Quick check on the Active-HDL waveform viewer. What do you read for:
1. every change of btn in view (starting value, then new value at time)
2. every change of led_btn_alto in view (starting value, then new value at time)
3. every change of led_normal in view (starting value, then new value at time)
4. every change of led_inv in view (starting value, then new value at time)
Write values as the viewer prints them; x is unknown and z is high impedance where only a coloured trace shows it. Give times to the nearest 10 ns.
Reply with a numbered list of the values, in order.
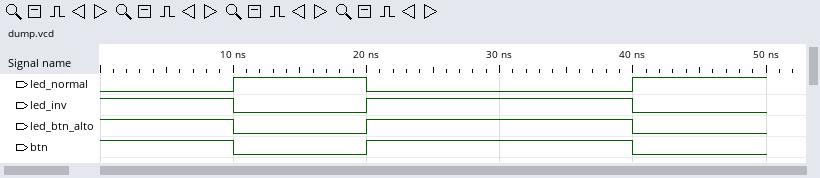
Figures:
1. 1, 0 at 10 ns, 1 at 20 ns, 0 at 40 ns
2. 1, 0 at 10 ns, 1 at 20 ns, 0 at 40 ns
3. 0, 1 at 10 ns, 0 at 20 ns, 1 at 40 ns
4. 1, 0 at 10 ns, 1 at 20 ns, 0 at 40 ns
